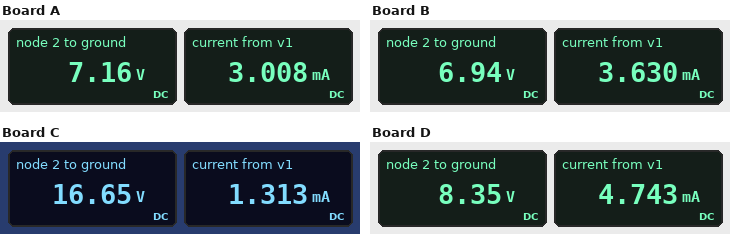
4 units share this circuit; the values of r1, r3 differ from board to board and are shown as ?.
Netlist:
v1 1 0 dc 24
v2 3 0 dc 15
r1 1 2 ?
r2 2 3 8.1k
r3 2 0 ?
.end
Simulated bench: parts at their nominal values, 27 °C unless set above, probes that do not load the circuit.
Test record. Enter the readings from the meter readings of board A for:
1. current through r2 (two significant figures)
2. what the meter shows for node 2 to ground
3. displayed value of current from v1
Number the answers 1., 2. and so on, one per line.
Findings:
1. 970 µA
2. 7.16 V
3. 3.008 mA
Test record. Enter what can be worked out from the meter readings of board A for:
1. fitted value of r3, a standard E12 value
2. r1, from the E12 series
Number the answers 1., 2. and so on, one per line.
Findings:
1. 1.8 kΩ
2. 5.6 kΩ
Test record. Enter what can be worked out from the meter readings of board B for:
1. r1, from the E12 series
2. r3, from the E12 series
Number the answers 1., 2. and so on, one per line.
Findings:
1. 4.7 kΩ
2. 1.5 kΩ
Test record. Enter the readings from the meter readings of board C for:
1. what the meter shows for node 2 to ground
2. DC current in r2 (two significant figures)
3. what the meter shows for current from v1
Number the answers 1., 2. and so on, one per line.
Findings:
1. 16.65 V
2. 200 µA
3. 1.313 mA
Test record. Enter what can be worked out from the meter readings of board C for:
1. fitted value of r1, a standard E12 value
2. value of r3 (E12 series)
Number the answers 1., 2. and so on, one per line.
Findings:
1. 5.6 kΩ
2. 15 kΩ
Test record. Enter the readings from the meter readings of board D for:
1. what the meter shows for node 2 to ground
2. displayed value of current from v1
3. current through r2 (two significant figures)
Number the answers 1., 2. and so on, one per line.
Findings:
1. 8.35 V
2. 4.743 mA
3. 820 µA
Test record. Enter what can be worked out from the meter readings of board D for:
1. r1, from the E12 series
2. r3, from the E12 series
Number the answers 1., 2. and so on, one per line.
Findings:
1. 3.3 kΩ
2. 1.5 kΩ
